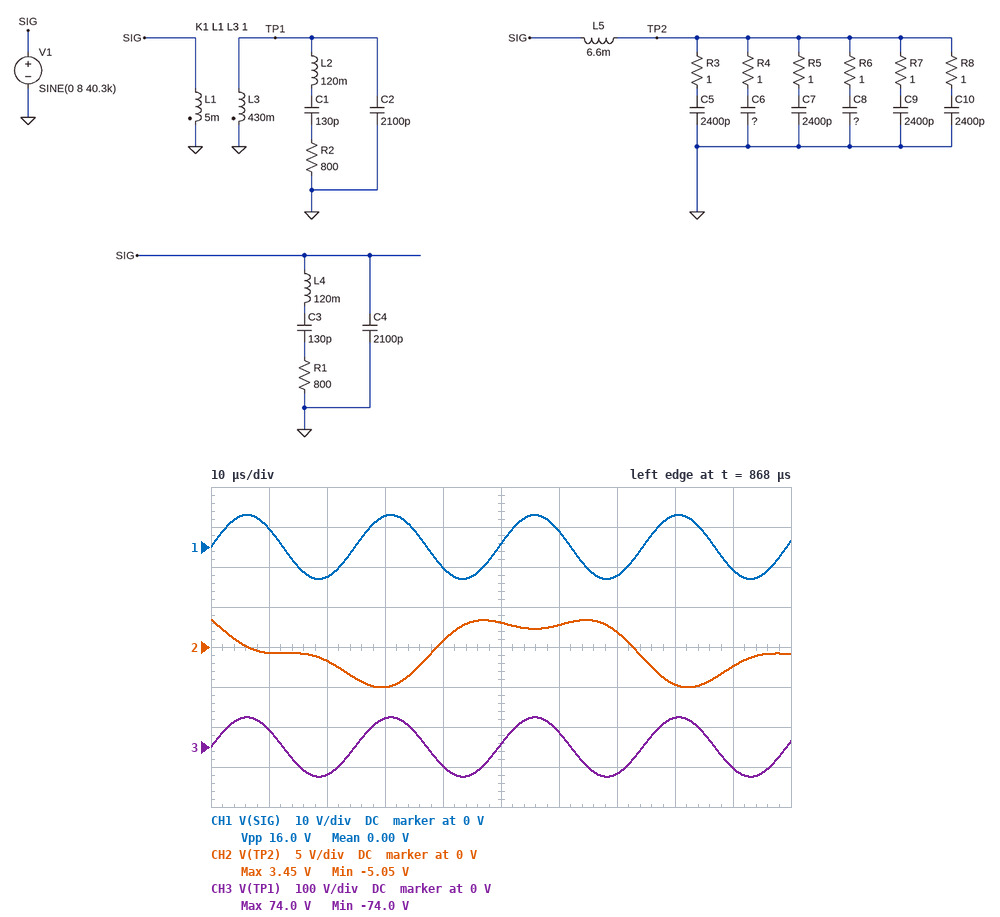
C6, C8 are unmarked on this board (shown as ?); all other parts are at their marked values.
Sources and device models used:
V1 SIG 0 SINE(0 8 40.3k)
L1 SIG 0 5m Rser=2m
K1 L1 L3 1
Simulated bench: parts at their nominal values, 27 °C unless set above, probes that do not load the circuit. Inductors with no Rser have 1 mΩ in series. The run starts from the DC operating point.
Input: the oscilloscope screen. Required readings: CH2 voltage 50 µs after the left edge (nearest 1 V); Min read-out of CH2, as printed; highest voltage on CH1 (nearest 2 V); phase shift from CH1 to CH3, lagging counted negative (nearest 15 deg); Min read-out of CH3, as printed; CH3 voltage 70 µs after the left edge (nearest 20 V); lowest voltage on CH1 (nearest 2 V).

3 V
-5.05 V
8 V
0 deg
-74.0 V
-60 V
-8 V
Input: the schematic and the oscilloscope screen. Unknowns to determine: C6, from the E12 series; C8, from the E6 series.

1.2 nF
3.3 nF
